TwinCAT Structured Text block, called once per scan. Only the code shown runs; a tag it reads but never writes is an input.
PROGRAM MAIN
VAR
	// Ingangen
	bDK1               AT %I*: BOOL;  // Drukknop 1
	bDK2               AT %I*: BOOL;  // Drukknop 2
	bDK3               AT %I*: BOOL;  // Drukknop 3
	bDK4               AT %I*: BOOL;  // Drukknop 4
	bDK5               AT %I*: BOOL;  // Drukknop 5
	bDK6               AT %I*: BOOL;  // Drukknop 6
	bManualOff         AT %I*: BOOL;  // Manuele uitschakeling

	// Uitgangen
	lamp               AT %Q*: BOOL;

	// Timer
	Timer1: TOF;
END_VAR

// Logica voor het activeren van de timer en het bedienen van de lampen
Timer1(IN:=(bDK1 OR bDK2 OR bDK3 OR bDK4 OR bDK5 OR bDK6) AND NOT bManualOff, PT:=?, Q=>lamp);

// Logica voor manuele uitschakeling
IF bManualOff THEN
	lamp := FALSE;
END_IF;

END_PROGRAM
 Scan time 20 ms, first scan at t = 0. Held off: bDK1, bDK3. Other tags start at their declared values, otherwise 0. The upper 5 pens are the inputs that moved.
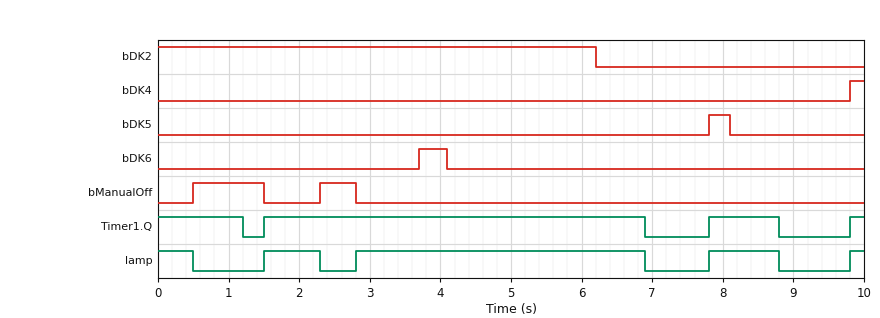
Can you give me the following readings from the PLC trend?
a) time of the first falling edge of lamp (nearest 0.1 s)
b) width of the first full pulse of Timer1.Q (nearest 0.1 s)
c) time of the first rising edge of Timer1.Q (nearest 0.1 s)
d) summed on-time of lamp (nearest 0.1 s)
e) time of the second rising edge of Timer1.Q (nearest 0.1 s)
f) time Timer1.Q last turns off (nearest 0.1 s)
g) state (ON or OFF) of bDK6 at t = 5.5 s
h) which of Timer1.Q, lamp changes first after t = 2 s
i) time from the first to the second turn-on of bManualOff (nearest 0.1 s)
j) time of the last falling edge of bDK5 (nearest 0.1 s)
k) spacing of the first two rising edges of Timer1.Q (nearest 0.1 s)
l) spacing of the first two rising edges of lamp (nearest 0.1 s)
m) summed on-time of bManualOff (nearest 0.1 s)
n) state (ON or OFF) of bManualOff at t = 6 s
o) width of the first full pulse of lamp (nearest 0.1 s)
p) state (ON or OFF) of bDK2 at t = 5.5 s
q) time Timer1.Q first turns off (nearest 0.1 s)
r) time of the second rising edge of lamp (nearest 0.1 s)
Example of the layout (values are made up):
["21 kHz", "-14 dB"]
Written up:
["0.5 s", "5.4 s", "1.5 s", "6.6 s", "7.8 s", "8.8 s", "OFF", "lamp", "1.8 s", "8.1 s", "6.3 s", "1.3 s", "1.5 s", "OFF", "0.8 s", "ON", "1.2 s", "2.8 s"]
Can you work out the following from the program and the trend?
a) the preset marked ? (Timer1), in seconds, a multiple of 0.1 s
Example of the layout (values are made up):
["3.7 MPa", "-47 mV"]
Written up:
["0.7 s"]
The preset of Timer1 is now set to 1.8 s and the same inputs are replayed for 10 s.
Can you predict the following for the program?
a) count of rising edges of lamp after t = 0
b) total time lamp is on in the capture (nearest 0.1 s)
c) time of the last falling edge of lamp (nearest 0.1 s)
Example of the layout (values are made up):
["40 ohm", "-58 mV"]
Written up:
["2", "8.5 s", "2.3 s"]
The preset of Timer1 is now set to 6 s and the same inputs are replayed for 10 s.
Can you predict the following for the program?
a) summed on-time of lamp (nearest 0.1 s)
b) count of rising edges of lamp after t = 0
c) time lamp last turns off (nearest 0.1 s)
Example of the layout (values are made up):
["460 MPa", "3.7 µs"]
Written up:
["8.5 s", "2", "2.3 s"]
